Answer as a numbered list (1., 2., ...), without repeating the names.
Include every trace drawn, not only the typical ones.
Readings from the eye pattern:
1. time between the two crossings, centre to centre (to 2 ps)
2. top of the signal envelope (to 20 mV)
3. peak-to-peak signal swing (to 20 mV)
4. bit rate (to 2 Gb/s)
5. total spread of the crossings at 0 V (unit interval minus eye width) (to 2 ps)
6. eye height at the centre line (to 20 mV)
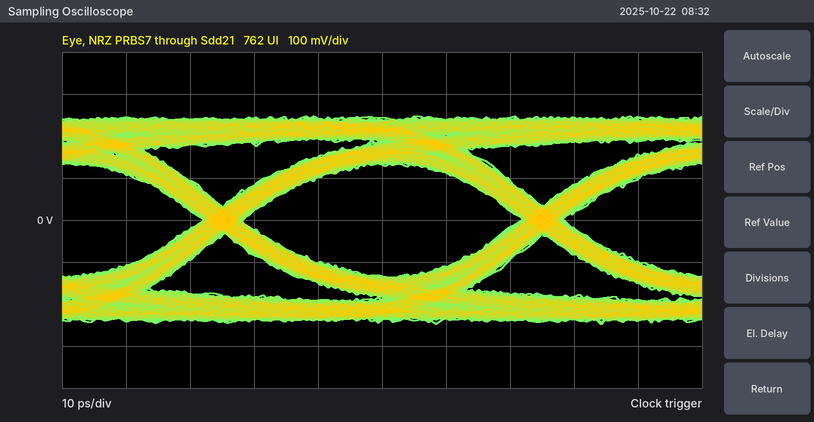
1. 50 ps
2. 240 mV
3. 500 mV
4. 20 Gb/s
5. 6 ps
6. 260 mV
